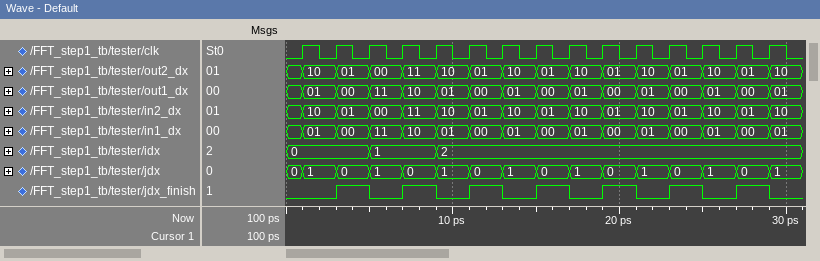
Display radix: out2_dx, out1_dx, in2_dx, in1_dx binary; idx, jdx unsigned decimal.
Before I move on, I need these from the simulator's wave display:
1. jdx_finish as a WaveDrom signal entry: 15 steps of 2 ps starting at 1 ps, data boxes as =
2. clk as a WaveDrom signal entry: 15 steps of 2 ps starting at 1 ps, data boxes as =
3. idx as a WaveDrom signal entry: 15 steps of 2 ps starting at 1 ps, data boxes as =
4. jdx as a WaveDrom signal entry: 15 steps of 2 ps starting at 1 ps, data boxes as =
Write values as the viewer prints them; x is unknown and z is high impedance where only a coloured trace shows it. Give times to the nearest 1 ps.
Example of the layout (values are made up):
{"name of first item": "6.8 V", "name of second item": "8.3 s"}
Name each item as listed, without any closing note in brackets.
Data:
{"jdx_finish as a WaveDrom signal entry: 15 steps of 2 ps starting at 1 ps, data boxes as =": "{name: 'jdx_finish', wave: '010101010101010'}", "clk as a WaveDrom signal entry: 15 steps of 2 ps starting at 1 ps, data boxes as =": "{name: 'clk', wave: 'p..............'}", "idx as a WaveDrom signal entry: 15 steps of 2 ps starting at 1 ps, data boxes as =": "{name: 'idx', wave: '=.=.=..........', data: '0 1 2'}", "jdx as a WaveDrom signal entry: 15 steps of 2 ps starting at 1 ps, data boxes as =": "{name: 'jdx', wave: '===============', data: '1 0 1 0 1 0 1 0 1 0 1 0 1 0 1'}"}
